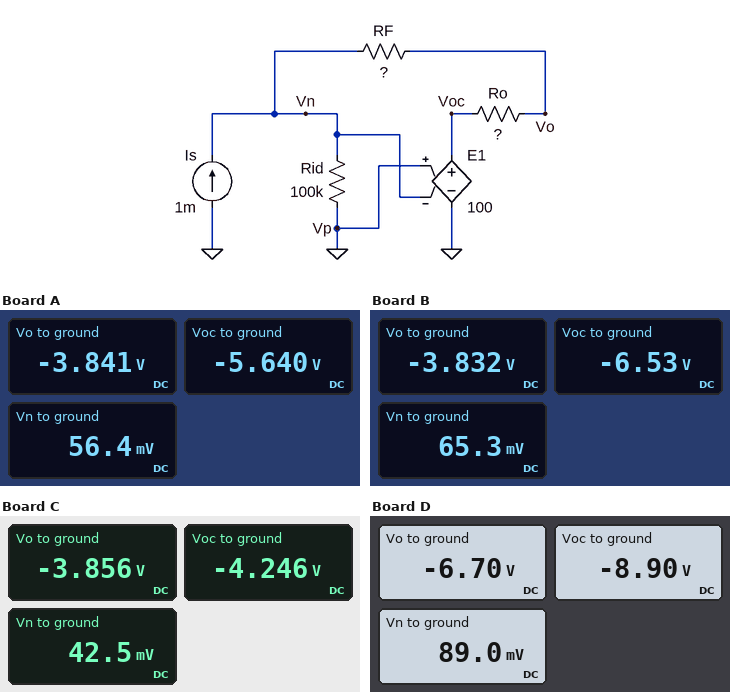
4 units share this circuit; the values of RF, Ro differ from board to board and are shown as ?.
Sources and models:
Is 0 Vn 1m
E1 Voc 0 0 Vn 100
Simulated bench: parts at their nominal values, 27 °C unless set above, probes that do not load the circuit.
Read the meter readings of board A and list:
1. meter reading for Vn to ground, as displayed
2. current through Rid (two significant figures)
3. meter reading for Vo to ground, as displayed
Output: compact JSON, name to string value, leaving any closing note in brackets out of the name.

{"meter reading for Vn to ground, as displayed": "56.4 mV", "current through Rid": "560 nA", "meter reading for Vo to ground, as displayed": "-3.841 V"}
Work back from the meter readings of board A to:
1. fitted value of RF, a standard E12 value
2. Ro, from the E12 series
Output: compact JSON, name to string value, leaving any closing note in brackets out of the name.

{"fitted value of RF, a standard E12 value": "3.9 kΩ", "Ro, from the E12 series": "1.8 kΩ"}
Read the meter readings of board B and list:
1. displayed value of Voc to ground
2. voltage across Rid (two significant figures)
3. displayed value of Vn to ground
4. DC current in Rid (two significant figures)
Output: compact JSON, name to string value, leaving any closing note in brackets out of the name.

{"displayed value of Voc to ground": "-6.53 V", "voltage across Rid": "65 mV", "displayed value of Vn to ground": "65.3 mV", "DC current in Rid": "650 nA"}
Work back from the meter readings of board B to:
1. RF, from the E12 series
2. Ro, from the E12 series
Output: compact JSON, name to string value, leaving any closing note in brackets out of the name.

{"RF, from the E12 series": "3.9 kΩ", "Ro, from the E12 series": "2.7 kΩ"}
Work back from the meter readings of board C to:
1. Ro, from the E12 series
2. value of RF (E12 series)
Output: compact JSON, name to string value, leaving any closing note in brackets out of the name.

{"Ro, from the E12 series": "390 Ω", "value of RF": "3.9 kΩ"}
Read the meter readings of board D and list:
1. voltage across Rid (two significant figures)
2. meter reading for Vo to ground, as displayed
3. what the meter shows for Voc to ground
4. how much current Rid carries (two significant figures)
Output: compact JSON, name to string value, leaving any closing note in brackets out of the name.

{"voltage across Rid": "89 mV", "meter reading for Vo to ground, as displayed": "-6.70 V", "what the meter shows for Voc to ground": "-8.90 V", "how much current Rid carries": "890 nA"}
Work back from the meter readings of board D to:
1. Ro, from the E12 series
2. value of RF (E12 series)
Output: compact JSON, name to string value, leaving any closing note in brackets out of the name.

{"Ro, from the E12 series": "2.2 kΩ", "value of RF": "6.8 kΩ"}
